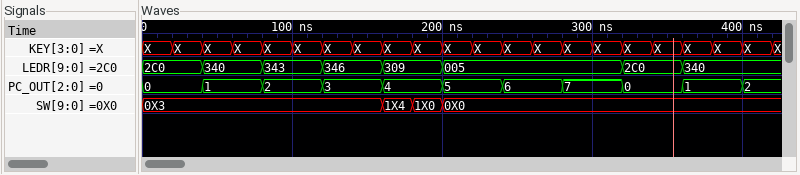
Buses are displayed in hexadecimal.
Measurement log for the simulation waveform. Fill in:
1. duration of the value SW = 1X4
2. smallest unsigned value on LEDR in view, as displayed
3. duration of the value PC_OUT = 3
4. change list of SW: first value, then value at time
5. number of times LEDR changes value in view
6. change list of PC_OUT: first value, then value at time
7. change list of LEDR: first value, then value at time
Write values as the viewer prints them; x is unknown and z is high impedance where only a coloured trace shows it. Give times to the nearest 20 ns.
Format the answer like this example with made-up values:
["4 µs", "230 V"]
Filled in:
["20 ns", "005", "40 ns", "0X3, 1X4 at 160 ns, 1X0 at 180 ns, 0X0 at 200 ns", "7", "0, 1 at 40 ns, 2 at 80 ns, 3 at 120 ns, 4 at 160 ns, 5 at 200 ns, 6 at 240 ns, 7 at 280 ns, 0 at 320 ns, 1 at 360 ns, 2 at 400 ns", "2C0, 340 at 40 ns, 343 at 80 ns, 346 at 120 ns, 309 at 160 ns, 005 at 200 ns, 2C0 at 320 ns, 340 at 360 ns"]
